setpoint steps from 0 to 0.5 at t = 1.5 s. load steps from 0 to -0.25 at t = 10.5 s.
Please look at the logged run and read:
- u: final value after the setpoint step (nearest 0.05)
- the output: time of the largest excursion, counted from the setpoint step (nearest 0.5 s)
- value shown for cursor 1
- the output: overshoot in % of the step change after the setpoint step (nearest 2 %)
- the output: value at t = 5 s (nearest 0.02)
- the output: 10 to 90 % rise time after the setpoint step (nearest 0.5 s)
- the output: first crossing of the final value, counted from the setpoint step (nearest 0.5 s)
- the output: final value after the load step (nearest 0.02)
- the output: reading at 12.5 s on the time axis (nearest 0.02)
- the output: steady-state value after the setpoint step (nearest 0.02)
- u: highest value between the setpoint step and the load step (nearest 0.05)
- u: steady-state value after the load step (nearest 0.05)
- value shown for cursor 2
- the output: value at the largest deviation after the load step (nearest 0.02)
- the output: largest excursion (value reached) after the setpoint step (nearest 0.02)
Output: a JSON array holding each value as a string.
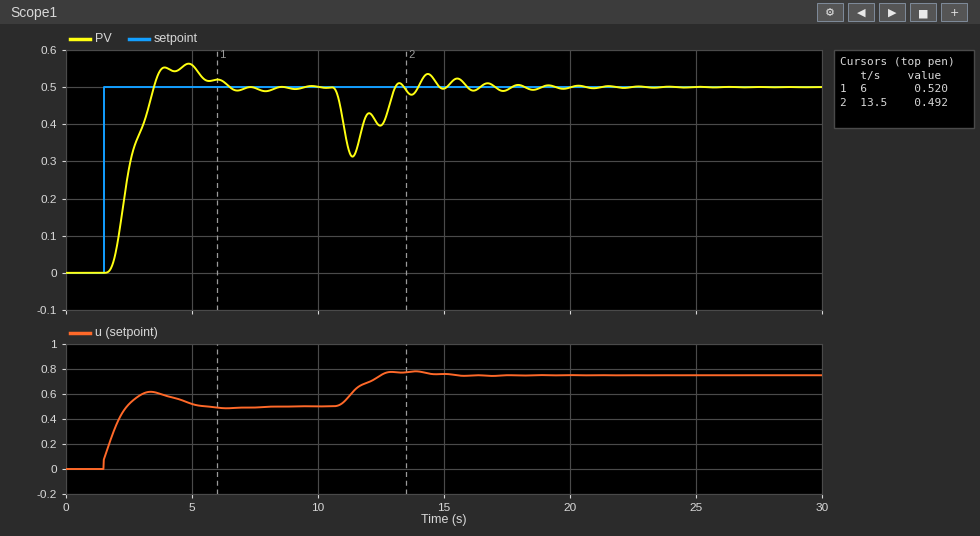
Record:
["0.50", "3.5 s", "0.520", "12 %", "0.56", "1.5 s", "2.0 s", "0.50", "0.40", "0.50", "0.60", "0.75", "0.492", "0.32", "0.56"]
